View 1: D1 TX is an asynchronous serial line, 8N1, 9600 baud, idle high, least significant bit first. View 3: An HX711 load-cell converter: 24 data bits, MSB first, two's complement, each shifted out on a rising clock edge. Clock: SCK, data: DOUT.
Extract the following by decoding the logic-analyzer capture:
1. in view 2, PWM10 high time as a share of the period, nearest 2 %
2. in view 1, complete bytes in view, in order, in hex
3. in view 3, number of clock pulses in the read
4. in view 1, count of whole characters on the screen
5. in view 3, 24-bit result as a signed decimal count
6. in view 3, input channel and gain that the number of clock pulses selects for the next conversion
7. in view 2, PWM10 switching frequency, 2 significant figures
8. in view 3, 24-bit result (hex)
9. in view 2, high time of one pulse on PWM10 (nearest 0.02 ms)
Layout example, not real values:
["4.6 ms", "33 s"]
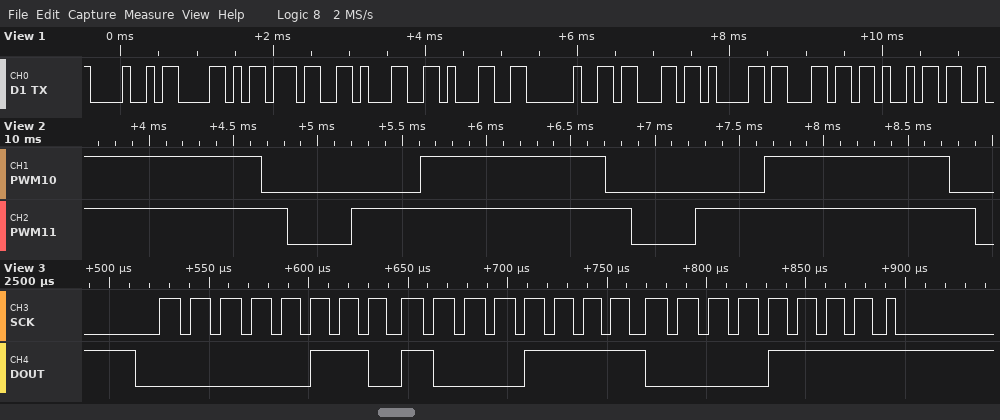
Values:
["54 %", "48 58 37 31 31 20 63 61 6C 69", "25", "10", "429839", "channel A, gain 128", "490 Hz", "0x068F0F", "1.10 ms"]
